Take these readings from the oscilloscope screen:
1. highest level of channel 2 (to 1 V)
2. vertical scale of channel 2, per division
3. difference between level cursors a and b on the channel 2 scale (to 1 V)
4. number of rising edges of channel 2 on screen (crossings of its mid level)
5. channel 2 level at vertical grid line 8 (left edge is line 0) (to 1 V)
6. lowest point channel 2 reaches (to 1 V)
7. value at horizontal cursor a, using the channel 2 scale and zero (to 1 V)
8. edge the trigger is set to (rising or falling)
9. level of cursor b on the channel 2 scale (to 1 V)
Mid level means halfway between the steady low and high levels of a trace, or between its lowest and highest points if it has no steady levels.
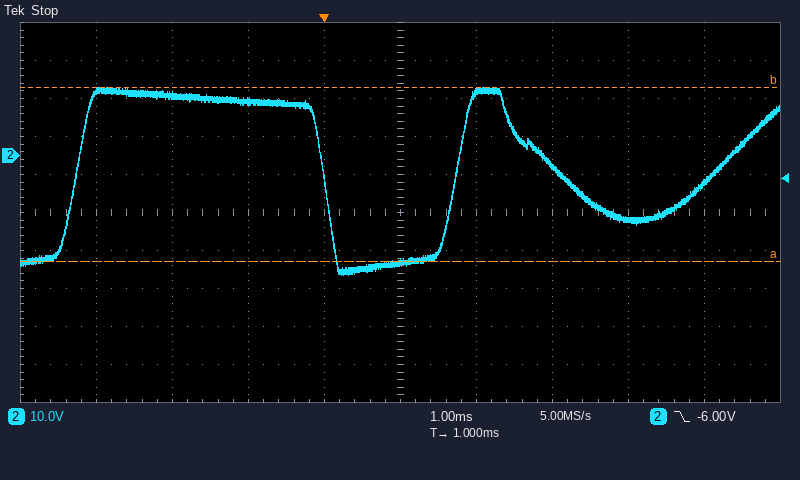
18 V
10 V
46 V
3
-17 V
-32 V
-28 V
falling
18 V
